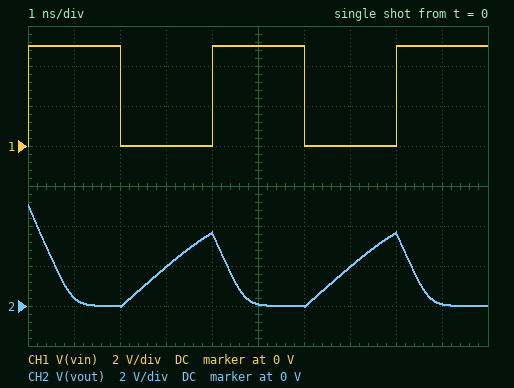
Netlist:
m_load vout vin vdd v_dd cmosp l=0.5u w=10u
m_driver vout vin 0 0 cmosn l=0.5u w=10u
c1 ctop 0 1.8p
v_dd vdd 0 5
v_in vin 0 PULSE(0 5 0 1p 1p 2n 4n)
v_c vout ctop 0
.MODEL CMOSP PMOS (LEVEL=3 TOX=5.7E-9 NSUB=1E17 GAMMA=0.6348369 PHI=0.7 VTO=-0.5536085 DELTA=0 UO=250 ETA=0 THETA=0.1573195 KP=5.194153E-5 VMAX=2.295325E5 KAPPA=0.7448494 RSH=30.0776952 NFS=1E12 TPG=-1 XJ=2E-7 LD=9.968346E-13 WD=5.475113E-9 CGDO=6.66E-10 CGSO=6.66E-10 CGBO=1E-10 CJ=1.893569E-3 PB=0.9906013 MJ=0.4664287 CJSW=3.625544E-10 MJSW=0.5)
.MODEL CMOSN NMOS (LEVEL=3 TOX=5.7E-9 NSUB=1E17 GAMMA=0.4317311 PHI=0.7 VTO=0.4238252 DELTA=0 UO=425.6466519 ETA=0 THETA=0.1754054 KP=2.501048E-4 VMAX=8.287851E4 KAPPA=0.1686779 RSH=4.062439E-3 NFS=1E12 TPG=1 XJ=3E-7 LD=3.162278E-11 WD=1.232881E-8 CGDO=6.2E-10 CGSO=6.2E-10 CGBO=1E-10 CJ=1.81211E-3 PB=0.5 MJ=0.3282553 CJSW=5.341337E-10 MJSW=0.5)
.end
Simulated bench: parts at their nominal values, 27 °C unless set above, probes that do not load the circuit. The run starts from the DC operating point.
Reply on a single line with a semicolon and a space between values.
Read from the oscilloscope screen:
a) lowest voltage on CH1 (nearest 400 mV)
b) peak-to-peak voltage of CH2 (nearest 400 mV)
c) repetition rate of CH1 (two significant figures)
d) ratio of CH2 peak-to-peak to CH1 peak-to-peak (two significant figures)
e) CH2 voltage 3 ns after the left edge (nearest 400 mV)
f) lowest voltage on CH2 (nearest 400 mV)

0 V; 5.2 V; 250 MHz; 1.0; 2.0 V; 0 V
